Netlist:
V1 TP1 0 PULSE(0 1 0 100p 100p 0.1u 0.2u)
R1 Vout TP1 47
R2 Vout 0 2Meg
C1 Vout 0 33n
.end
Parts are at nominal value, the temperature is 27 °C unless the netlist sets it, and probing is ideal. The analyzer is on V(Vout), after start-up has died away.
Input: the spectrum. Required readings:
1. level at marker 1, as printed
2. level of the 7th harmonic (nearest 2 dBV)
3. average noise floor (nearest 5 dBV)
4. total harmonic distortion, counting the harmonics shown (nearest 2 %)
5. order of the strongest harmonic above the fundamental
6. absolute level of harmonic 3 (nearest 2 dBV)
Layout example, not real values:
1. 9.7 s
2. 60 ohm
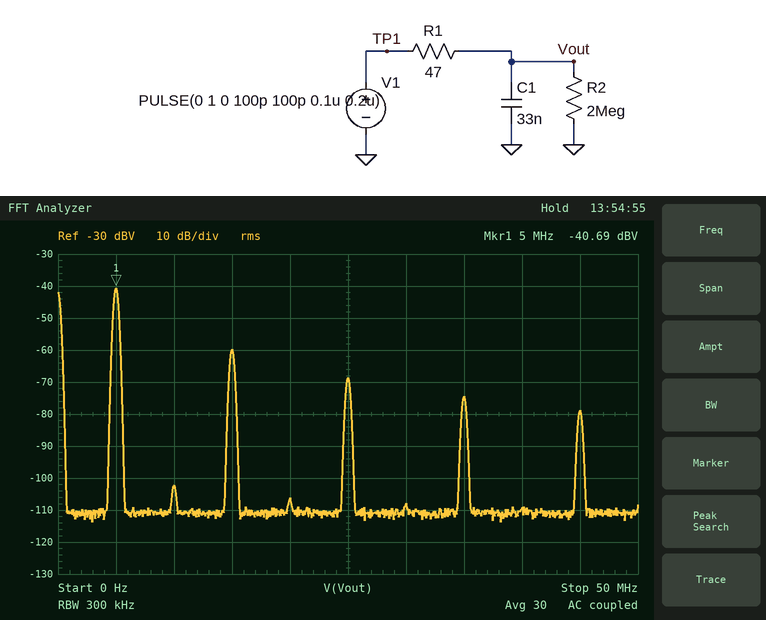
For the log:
1. -40.69 dBV
2. -74 dBV
3. -110 dBV
4. 12 %
5. 3
6. -60 dBV
